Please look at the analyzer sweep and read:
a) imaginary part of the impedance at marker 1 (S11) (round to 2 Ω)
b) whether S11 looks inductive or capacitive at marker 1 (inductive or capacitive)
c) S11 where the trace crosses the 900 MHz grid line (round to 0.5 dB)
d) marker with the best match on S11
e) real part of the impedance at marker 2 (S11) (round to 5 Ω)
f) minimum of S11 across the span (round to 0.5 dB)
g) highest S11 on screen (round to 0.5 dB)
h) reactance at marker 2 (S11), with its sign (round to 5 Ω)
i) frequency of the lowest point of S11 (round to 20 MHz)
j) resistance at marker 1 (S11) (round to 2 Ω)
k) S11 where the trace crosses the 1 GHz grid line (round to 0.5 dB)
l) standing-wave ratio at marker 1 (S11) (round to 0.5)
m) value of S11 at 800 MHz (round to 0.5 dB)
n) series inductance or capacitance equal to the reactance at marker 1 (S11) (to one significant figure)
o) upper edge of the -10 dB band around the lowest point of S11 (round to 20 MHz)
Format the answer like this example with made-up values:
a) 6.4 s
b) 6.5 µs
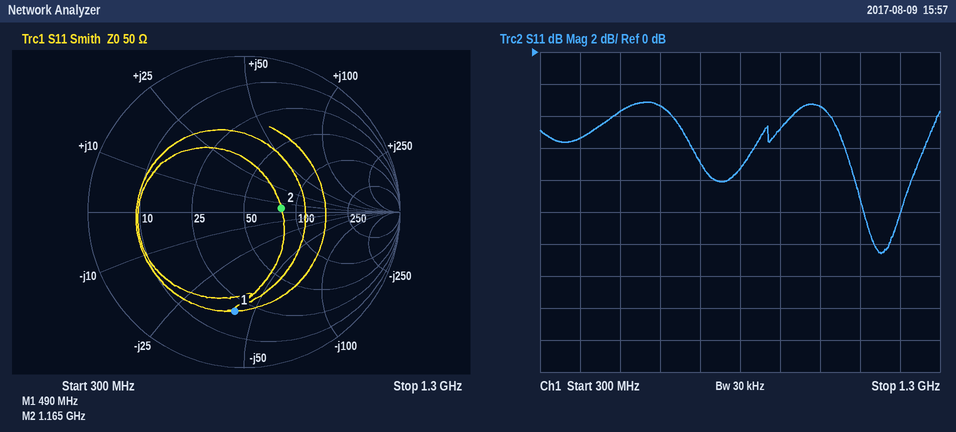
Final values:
a) -42 Ω
b) capacitive
c) -5.0 dB
d) marker 2
e) 80 Ω
f) -12.5 dB
g) -3.0 dB
h) +5 Ω
i) 1.16 GHz
j) 20 Ω
k) -3.5 dB
l) 4.5
m) -7.5 dB
n) 8 pF
o) 1.20 GHz
